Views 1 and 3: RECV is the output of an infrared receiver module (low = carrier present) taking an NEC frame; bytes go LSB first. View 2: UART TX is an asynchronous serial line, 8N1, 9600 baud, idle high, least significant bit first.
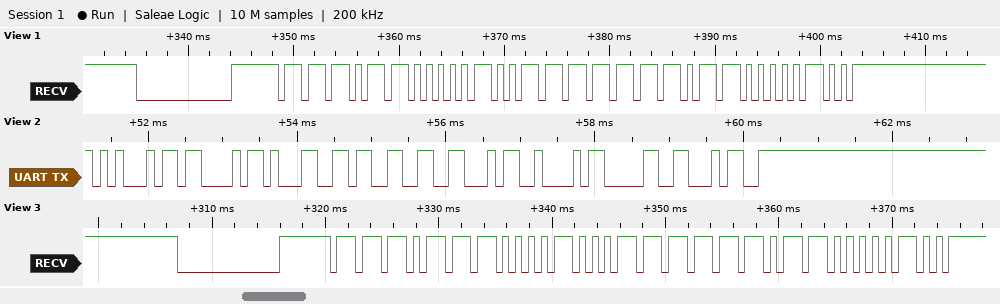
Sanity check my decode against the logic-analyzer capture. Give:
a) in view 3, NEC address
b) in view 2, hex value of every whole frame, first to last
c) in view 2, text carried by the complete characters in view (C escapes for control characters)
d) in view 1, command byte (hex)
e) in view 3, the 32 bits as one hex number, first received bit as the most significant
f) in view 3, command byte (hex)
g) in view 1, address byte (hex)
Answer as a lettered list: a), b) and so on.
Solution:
a) 0x77
b) 0x45 0x43 0x31 0x33 0x46 0x42 0x30 0x34
c) "EC13FB04"
d) 0xDF
e) 0xEE11FB04
f) 0xDF
g) 0x37
